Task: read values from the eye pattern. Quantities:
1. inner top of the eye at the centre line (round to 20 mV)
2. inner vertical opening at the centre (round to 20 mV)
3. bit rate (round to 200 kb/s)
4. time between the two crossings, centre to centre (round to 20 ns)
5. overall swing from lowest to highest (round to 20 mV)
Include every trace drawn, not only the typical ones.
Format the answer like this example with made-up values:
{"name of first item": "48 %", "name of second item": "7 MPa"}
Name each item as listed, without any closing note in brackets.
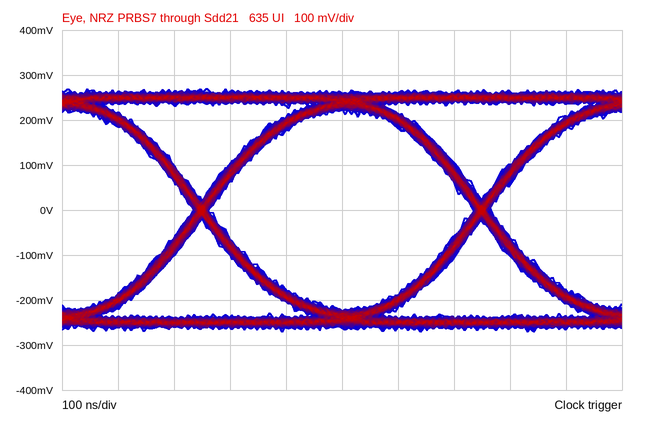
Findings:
{"inner top of the eye at the centre line": "220 mV", "inner vertical opening at the centre": "440 mV", "bit rate": "2.0 Mb/s", "time between the two crossings, centre to centre": "500 ns", "overall swing from lowest to highest": "540 mV"}
